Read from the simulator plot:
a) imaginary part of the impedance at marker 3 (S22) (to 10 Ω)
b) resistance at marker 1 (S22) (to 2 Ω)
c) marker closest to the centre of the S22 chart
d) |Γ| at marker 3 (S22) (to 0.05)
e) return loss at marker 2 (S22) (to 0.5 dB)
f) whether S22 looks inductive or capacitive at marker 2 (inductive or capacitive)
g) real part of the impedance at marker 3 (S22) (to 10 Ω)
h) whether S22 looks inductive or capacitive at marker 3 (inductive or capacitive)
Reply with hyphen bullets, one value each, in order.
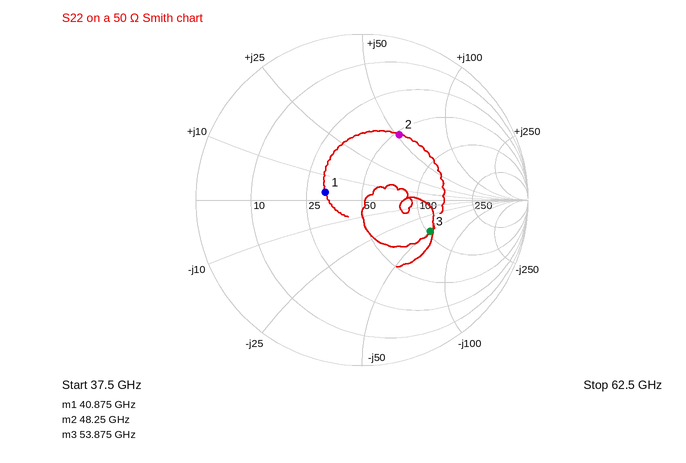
- -50 Ω
- 32 Ω
- marker 1
- 0.45
- 7.0 dB
- inductive
- 100 Ω
- capacitive
